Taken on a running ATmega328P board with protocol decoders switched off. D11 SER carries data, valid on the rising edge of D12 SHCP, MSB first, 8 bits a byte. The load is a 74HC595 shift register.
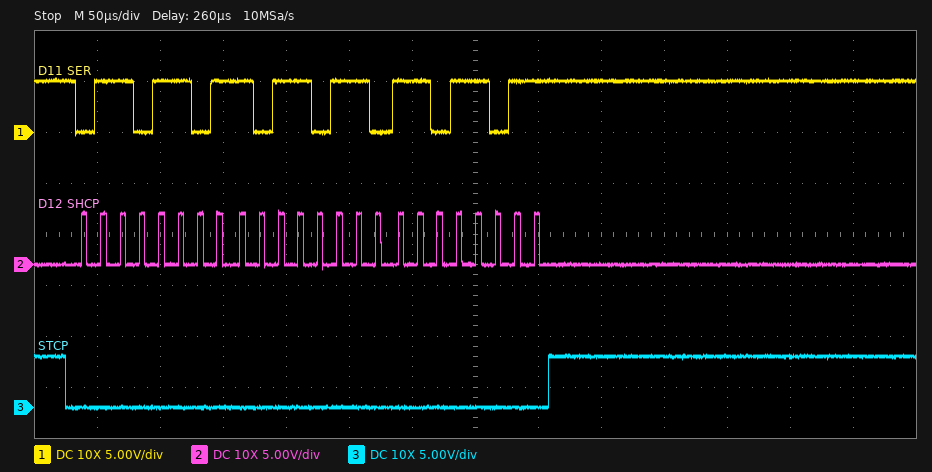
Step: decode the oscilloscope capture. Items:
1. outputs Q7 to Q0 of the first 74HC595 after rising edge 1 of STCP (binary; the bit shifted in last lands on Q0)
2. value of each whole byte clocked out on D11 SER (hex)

11011011
6D B6 DB
